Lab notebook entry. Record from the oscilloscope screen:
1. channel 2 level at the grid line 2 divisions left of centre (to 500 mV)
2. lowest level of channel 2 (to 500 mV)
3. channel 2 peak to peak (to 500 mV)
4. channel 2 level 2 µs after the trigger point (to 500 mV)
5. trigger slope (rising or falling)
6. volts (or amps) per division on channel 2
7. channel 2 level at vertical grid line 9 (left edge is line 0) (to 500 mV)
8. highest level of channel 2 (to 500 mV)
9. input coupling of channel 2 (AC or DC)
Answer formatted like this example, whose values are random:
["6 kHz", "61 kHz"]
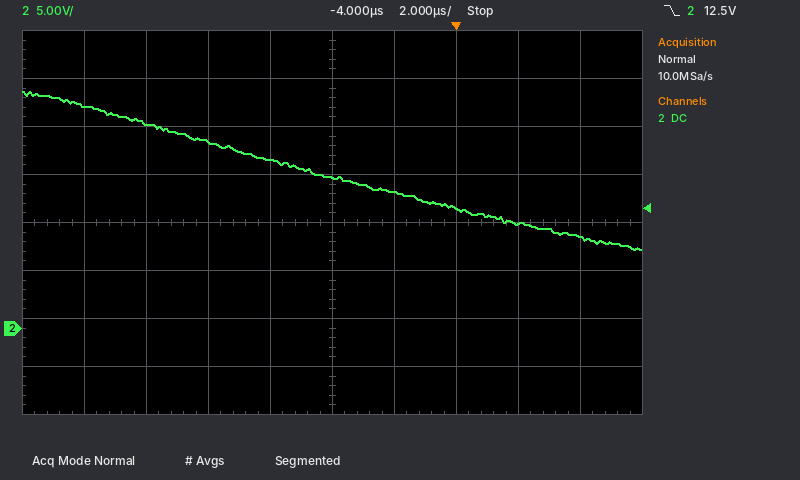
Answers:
["19.5 V", "8.0 V", "16.5 V", "11.0 V", "falling", "5 V", "9.5 V", "24.5 V", "DC"]
